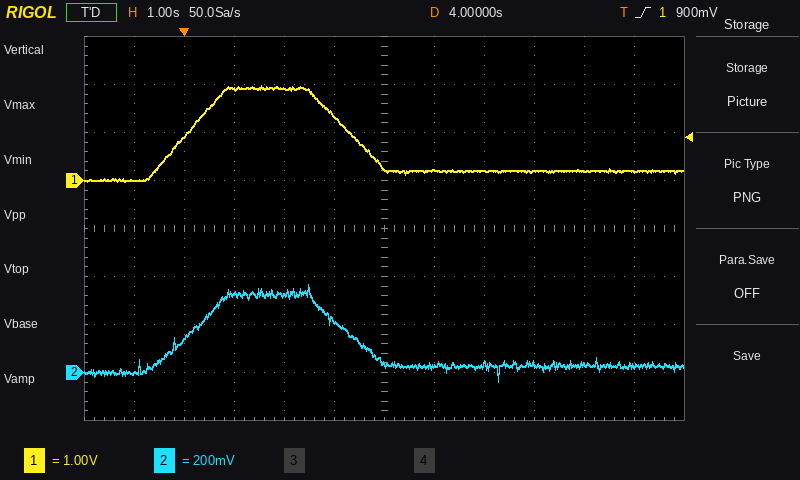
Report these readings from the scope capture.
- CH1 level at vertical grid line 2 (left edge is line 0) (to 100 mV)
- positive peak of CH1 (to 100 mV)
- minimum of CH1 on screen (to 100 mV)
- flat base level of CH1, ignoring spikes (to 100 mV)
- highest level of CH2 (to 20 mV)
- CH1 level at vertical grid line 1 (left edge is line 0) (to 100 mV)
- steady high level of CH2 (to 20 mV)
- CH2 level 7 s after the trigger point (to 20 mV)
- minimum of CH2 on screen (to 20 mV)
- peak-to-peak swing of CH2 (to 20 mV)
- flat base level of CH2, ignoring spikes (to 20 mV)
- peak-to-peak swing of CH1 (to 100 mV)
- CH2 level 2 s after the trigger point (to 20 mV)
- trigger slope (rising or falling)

900 mV
2.0 V
0.0 V
200 mV
360 mV
0.0 V
320 mV
40 mV
-40 mV
400 mV
20 mV
2.0 V
320 mV
rising
